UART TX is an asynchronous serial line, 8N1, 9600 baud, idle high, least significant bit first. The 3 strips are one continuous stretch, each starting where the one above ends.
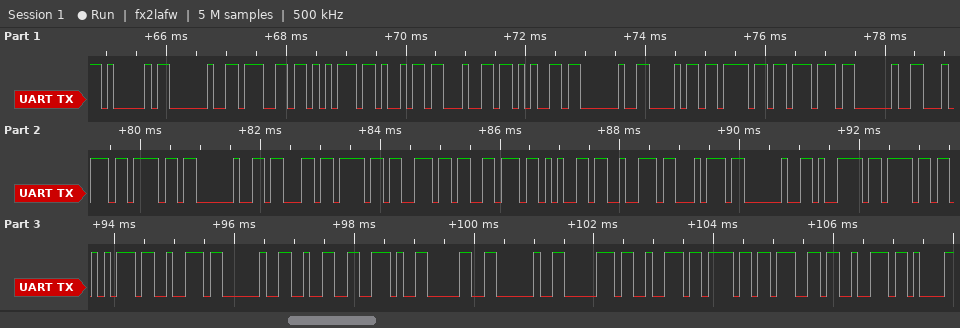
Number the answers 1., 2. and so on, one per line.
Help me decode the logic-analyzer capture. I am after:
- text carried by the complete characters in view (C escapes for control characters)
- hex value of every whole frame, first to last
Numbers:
1. "A guide how to convert your 2.0 progr"
2. 0x41 0x20 0x67 0x75 0x69 0x64 0x65 0x20 0x68 0x6F 0x77 0x20 0x74 0x6F 0x20 0x63 0x6F 0x6E 0x76 0x65 0x72 0x74 0x20 0x79 0x6F 0x75 0x72 0x20 0x32 0x2E 0x30 0x20 0x70 0x72 0x6F 0x67 0x72
